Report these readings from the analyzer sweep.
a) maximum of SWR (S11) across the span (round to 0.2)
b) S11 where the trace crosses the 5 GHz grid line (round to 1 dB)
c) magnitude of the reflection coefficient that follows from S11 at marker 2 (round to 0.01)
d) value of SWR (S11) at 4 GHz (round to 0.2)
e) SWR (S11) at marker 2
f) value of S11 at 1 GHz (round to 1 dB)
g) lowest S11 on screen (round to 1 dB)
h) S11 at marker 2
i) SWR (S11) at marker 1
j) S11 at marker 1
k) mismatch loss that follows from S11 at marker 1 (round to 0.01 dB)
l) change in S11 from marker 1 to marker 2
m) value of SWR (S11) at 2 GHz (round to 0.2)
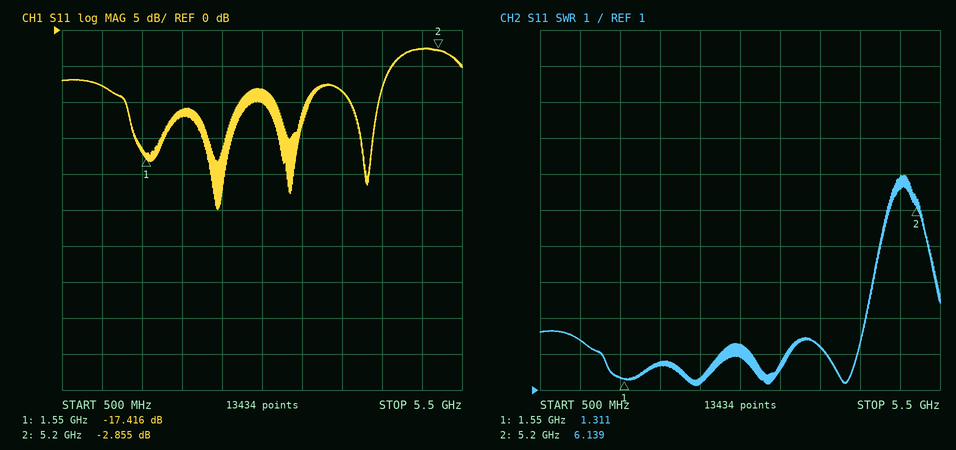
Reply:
7.0
-3 dB
0.72
2.2
6.139
-8 dB
-25 dB
-2.855 dB
1.311
-17.416 dB
0.08 dB
14.561 dB
1.8
